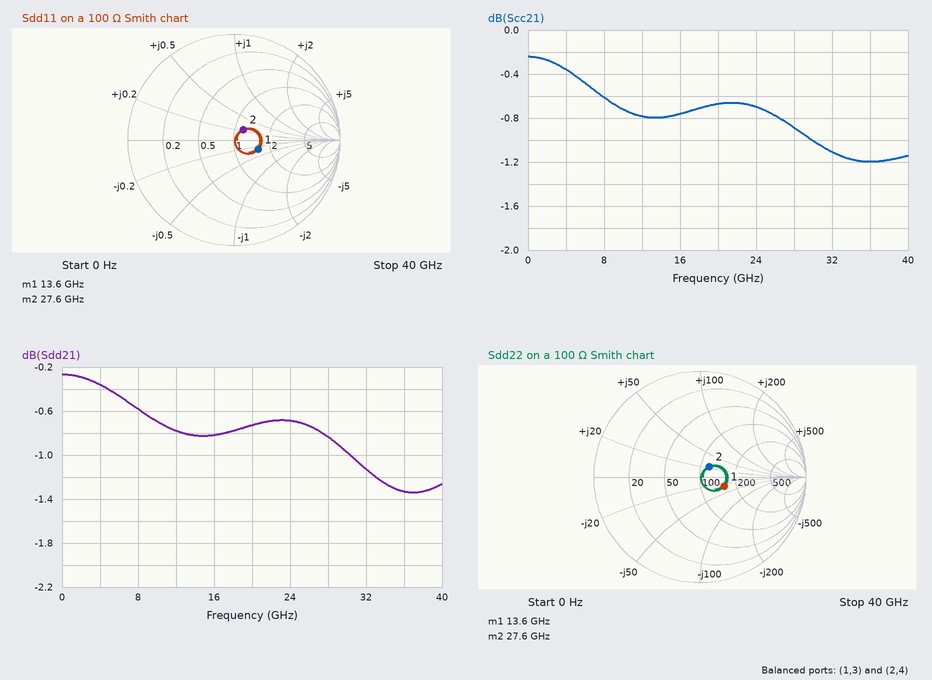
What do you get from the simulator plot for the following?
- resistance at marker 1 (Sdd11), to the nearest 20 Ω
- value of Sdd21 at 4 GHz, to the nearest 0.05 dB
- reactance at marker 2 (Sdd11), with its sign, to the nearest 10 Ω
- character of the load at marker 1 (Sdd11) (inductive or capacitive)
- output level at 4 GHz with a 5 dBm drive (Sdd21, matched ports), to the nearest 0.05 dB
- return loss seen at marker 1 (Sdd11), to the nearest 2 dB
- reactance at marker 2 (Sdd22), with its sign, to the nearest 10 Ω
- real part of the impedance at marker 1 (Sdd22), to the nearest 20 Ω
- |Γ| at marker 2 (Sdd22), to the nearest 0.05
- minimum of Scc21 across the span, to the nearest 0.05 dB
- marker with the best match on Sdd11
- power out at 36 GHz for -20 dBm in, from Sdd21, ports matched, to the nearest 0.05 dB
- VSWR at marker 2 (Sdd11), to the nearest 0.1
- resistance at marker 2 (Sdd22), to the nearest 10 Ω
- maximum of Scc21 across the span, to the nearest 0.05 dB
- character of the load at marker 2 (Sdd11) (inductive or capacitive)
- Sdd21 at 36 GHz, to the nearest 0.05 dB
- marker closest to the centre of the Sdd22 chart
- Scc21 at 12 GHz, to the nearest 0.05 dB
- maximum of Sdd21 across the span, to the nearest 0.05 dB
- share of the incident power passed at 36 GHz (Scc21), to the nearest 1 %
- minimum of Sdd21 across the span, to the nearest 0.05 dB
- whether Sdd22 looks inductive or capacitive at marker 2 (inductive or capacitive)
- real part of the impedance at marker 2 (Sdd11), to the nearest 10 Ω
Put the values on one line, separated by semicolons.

160 Ω; -0.35 dB; +20 Ω; capacitive; 4.65 dBm; 12 dB; +20 Ω; 160 Ω; 0.15; -1.20 dB; marker 2; -21.35 dBm; 1.3; 120 Ω; -0.25 dB; inductive; -1.35 dB; marker 2; -0.80 dB; -0.25 dB; 76 %; -1.35 dB; inductive; 120 Ω
